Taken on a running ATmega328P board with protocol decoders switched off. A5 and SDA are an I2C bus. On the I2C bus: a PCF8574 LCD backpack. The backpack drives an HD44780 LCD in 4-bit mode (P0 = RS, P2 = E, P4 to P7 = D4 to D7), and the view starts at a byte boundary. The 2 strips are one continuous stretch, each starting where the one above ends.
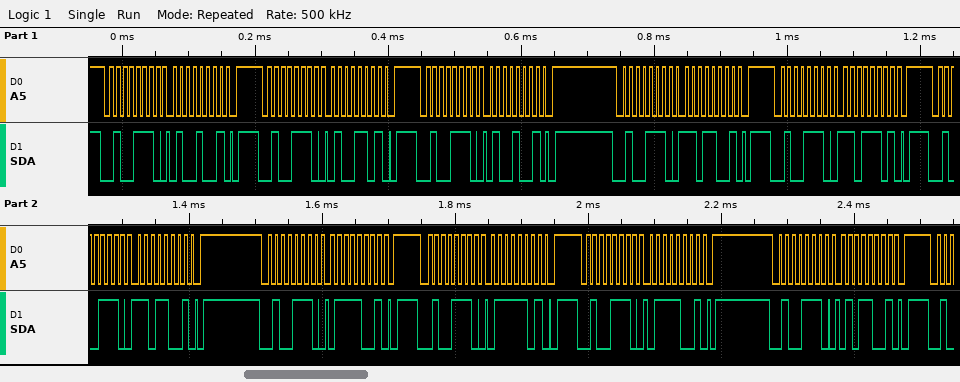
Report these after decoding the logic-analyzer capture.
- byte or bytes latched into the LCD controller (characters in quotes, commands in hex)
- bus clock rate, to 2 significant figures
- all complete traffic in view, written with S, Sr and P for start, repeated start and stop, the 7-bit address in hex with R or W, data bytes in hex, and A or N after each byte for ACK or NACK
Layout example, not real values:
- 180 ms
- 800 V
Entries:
- 'M'
- 100 kHz
- S 27W A 49 A P S 27W A 4D A P S 27W A 49 A P S 27W A D9 A P S 27W A DD A P S 27W A D9 A P S 27W A 79 A P S 27W A 7D A P S 27W A 79 A P S 27W A 59 A P
